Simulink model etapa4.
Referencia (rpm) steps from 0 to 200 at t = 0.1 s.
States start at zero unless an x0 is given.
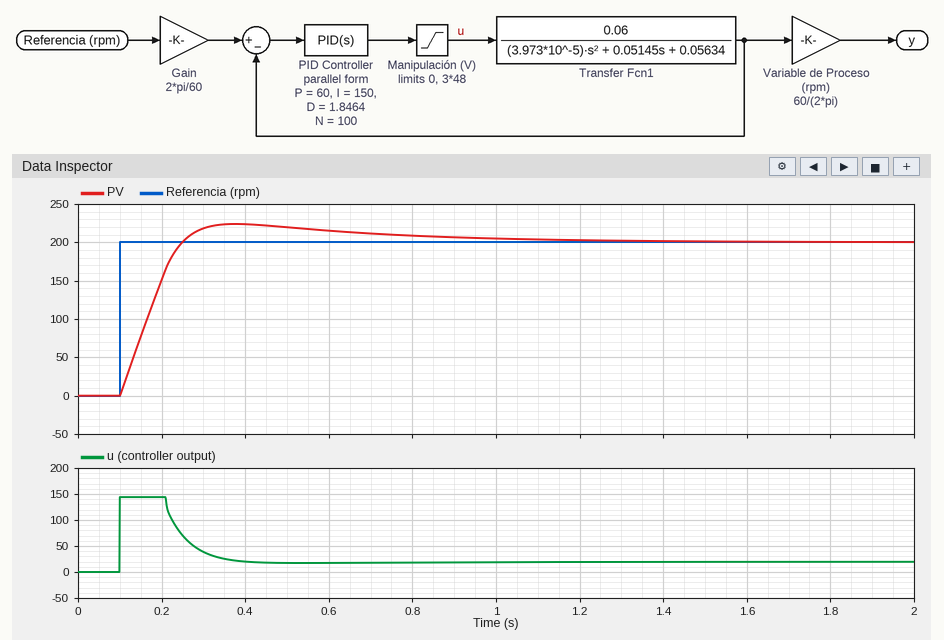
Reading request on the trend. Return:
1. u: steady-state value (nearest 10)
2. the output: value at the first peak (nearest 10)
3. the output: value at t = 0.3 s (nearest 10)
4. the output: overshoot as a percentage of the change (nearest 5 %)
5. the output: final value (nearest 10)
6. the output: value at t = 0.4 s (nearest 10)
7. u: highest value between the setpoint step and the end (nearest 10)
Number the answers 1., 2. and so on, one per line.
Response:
1. 20
2. 220
3. 220
4. 10 %
5. 200
6. 220
7. 140
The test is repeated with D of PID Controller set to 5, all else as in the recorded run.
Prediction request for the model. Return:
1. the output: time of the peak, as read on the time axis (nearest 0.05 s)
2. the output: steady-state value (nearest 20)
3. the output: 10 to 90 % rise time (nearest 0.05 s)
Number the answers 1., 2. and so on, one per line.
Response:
1. 0.50 s
2. 200
3. 0.15 s
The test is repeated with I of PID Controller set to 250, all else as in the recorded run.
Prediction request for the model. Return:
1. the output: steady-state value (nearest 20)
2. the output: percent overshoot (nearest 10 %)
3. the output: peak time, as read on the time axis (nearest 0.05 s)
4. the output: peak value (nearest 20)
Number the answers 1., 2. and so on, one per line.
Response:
1. 200
2. 20 %
3. 0.35 s
4. 240
